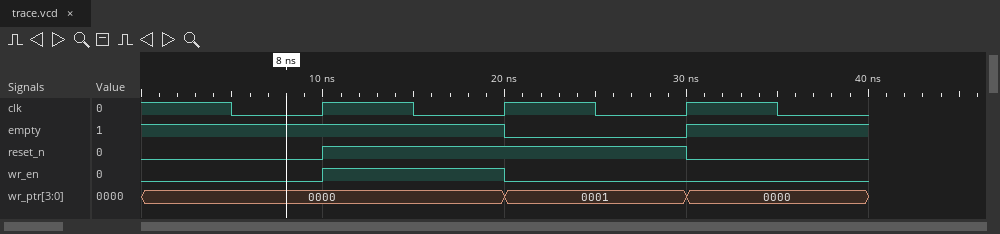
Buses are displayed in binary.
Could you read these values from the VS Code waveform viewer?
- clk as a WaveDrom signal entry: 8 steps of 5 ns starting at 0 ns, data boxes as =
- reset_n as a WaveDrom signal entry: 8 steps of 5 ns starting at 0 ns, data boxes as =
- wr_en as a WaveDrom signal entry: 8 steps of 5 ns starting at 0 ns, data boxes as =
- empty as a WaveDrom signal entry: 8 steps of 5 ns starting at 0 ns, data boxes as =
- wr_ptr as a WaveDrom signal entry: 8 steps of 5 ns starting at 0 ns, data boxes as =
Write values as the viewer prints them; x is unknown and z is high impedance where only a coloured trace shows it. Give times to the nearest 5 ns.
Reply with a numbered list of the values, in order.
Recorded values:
1. {name: 'clk', wave: '10101010'}
2. {name: 'reset_n', wave: '0.1...0.'}
3. {name: 'wr_en', wave: '0.1.0...'}
4. {name: 'empty', wave: '1...0.1.'}
5. {name: 'wr_ptr', wave: '=...=.=.', data: '0000 0001 0000'}
